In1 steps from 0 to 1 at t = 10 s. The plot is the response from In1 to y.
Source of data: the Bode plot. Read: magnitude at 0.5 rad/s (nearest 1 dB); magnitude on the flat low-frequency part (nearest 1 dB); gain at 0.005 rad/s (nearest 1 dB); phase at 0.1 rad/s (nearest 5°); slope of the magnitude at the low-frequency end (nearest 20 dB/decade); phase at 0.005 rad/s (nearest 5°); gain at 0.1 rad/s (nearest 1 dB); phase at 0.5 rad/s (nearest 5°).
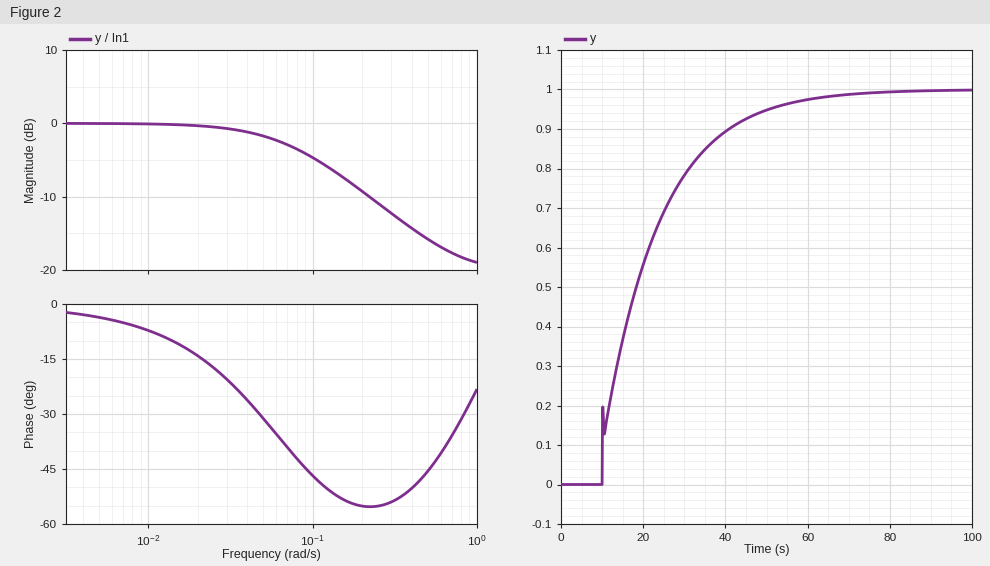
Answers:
-16 dB
0 dB
0 dB
-45°
0 dB/decade
-5°
-5 dB
-45°
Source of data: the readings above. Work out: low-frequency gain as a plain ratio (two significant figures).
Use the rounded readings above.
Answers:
1.0
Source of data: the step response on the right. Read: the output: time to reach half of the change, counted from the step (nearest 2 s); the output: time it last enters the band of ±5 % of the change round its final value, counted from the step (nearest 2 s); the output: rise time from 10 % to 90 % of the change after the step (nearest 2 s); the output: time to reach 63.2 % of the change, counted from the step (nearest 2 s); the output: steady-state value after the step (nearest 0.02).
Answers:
8 s
40 s
30 s
12 s
1.00
